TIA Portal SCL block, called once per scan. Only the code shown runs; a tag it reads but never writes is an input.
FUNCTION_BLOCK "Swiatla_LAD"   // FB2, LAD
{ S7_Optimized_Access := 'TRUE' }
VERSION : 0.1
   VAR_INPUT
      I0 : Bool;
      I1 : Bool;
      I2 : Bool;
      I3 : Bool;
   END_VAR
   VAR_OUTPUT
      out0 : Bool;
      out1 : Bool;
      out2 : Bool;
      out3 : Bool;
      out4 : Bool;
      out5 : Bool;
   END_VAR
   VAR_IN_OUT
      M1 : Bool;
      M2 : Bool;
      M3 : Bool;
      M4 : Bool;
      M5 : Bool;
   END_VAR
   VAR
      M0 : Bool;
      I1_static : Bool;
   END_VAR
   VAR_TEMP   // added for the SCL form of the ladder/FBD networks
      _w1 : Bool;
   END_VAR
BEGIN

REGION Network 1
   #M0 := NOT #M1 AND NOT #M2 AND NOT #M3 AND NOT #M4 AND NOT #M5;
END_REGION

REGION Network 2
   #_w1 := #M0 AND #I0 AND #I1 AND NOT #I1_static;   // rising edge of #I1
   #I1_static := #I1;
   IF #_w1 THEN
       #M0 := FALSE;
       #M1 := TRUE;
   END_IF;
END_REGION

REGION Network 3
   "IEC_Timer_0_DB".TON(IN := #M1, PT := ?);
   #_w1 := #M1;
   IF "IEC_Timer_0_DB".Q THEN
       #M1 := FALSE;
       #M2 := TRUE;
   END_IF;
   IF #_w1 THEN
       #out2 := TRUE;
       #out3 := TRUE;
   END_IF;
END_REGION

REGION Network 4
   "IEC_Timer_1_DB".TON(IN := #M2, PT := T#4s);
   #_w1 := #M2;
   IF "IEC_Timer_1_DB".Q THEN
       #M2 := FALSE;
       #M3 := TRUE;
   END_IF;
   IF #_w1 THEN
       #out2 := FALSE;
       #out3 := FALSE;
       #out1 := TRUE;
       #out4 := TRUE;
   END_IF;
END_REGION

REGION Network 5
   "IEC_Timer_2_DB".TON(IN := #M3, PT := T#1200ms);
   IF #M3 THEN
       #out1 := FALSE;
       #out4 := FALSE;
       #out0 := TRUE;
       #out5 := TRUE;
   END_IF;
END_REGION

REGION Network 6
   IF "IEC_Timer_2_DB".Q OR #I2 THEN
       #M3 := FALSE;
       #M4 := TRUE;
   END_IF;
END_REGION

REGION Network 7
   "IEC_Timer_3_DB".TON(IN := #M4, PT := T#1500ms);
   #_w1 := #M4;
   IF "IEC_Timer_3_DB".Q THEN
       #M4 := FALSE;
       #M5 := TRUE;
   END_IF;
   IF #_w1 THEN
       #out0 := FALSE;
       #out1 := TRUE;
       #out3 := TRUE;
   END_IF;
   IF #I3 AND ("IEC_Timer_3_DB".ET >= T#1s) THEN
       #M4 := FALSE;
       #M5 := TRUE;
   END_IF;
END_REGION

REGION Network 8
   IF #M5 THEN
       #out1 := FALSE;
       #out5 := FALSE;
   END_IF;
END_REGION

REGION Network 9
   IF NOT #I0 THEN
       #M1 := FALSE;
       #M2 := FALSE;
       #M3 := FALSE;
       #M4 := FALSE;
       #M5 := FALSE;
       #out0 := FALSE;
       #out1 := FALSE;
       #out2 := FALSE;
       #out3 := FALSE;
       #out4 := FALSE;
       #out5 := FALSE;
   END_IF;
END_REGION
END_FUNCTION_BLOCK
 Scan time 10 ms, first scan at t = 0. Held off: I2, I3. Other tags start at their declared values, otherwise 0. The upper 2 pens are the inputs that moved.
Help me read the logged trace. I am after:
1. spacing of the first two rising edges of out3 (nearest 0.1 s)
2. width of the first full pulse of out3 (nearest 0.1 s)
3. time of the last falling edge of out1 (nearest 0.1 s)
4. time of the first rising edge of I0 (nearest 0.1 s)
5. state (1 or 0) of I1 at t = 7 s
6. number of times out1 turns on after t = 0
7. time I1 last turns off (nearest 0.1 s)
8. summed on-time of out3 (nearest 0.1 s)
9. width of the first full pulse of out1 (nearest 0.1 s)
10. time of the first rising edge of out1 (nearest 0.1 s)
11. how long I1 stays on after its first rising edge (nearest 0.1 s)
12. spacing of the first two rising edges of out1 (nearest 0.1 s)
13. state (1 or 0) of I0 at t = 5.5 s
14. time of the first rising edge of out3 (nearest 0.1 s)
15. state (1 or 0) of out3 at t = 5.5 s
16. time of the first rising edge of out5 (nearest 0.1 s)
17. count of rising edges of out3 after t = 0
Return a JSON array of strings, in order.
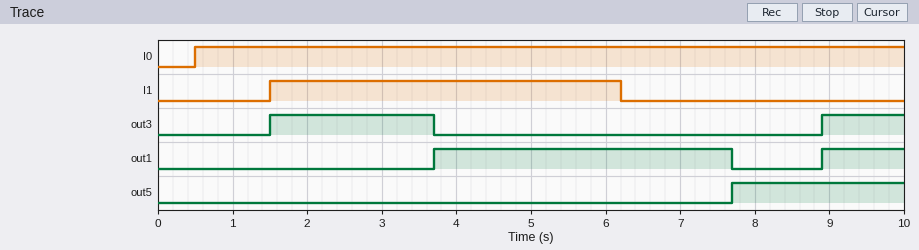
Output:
["7.4 s", "2.2 s", "7.7 s", "0.5 s", "0", "2", "6.2 s", "3.3 s", "4.0 s", "3.7 s", "4.7 s", "5.2 s", "1", "1.5 s", "0", "7.7 s", "2"]
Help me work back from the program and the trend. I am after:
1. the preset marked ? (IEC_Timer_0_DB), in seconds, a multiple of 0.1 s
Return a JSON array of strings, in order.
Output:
["2.2 s"]
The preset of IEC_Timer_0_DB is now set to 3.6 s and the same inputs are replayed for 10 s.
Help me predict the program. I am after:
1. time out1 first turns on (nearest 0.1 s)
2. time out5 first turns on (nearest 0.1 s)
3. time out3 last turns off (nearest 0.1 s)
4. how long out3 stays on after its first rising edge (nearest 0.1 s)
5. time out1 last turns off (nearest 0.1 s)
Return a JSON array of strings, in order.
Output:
["5.1 s", "9.1 s", "5.1 s", "3.6 s", "9.1 s"]
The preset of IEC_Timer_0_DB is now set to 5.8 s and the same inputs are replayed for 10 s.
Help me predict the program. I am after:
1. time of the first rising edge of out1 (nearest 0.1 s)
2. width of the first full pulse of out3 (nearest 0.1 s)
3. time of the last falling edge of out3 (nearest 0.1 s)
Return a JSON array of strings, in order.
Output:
["7.3 s", "5.8 s", "7.3 s"]
